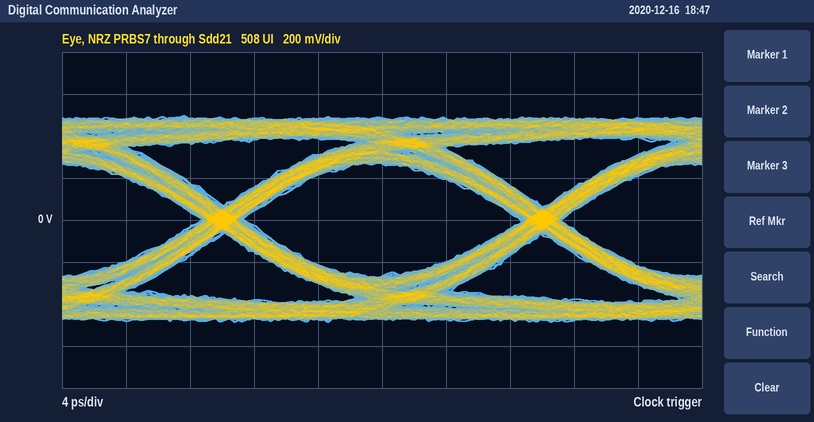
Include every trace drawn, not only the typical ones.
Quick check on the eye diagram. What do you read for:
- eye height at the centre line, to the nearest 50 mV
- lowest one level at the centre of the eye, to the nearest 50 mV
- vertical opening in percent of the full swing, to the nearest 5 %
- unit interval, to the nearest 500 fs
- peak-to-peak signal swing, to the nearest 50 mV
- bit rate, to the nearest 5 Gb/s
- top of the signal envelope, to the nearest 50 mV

550 mV
250 mV
55 %
20.0 ps
1.00 V
50 Gb/s
500 mV
